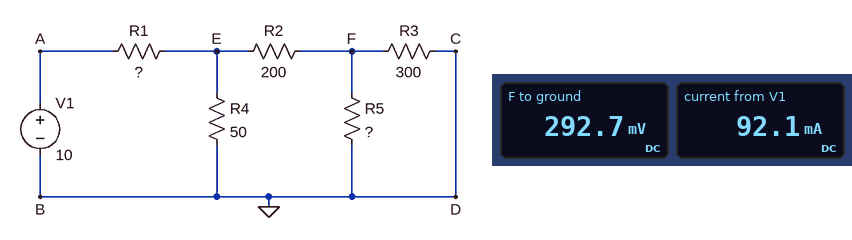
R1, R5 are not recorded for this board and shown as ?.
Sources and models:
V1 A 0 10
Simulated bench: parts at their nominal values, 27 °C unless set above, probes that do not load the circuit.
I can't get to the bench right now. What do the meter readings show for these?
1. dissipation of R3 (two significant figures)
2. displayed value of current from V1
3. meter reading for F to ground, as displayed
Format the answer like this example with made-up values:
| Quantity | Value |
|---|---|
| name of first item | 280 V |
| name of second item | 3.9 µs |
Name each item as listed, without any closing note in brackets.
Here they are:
| Quantity | Value |
|---|---|
| dissipation of R3 | 290 µW |
| displayed value of current from V1 | 92.1 mA |
| meter reading for F to ground, as displayed | 292.7 mV |
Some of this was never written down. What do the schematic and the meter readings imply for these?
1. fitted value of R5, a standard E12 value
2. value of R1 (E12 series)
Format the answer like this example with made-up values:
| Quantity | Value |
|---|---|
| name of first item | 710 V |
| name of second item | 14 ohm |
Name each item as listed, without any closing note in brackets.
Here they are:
| Quantity | Value |
|---|---|
| fitted value of R5, a standard E12 value | 18 Ω |
| value of R1 | 68 Ω |
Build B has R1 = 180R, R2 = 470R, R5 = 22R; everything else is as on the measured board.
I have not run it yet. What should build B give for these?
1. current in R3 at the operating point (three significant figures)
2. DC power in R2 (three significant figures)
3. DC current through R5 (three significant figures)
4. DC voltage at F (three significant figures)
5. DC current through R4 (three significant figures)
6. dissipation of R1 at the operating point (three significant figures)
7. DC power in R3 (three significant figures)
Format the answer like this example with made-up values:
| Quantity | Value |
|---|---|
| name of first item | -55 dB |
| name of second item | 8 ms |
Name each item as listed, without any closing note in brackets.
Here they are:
| Quantity | Value |
|---|---|
| current in R3 at the operating point | 280 µA |
| DC power in R2 | 7.92 mW |
| DC current through R5 | 3.82 mA |
| DC voltage at F | 84.1 mV |
| DC current through R4 | 40.3 mA |
| dissipation of R1 at the operating point | 354 mW |
| DC power in R3 | 23.6 µW |
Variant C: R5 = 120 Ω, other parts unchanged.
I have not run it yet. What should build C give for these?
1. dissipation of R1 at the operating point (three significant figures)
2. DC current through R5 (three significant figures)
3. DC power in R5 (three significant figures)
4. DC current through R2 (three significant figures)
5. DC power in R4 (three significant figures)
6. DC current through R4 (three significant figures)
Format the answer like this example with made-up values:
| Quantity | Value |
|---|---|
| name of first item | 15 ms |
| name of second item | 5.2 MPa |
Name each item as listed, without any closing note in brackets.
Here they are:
| Quantity | Value |
|---|---|
| dissipation of R1 at the operating point | 556 mW |
| DC current through R5 | 9.62 mA |
| DC power in R5 | 11.1 mW |
| DC current through R2 | 13.5 mA |
| DC power in R4 | 296 mW |
| DC current through R4 | 77.0 mA |
